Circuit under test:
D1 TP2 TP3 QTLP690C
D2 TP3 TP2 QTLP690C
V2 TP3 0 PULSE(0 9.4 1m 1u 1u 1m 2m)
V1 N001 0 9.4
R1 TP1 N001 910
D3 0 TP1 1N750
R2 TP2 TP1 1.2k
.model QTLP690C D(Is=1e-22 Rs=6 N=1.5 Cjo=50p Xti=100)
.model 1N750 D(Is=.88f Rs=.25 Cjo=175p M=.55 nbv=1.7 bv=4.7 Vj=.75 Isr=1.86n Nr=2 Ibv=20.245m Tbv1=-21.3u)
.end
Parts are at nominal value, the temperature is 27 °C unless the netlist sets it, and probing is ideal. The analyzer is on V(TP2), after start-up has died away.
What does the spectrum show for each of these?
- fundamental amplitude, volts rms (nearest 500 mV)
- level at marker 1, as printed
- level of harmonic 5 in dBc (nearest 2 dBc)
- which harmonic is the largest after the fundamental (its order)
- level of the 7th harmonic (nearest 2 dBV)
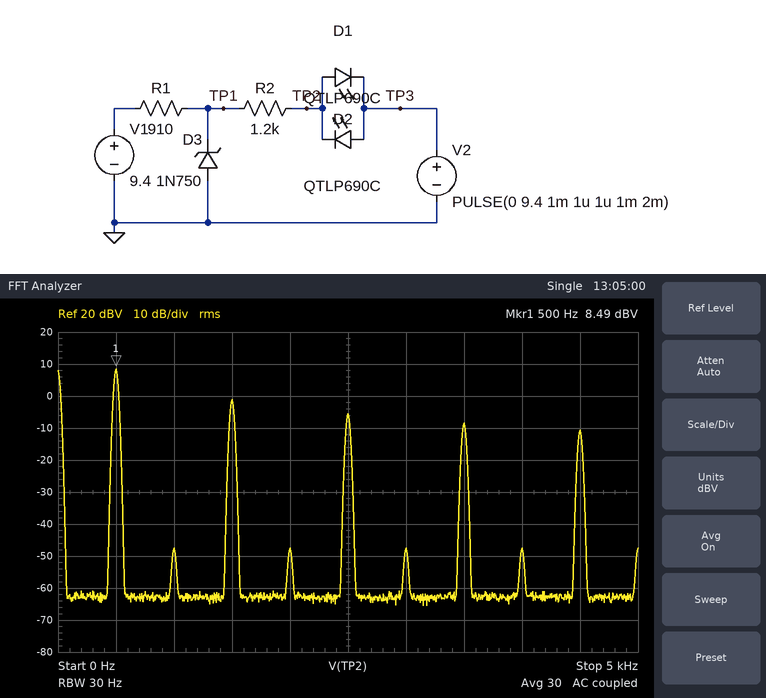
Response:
2.5 V
8.49 dBV
-14 dBc
3
-8 dBV
